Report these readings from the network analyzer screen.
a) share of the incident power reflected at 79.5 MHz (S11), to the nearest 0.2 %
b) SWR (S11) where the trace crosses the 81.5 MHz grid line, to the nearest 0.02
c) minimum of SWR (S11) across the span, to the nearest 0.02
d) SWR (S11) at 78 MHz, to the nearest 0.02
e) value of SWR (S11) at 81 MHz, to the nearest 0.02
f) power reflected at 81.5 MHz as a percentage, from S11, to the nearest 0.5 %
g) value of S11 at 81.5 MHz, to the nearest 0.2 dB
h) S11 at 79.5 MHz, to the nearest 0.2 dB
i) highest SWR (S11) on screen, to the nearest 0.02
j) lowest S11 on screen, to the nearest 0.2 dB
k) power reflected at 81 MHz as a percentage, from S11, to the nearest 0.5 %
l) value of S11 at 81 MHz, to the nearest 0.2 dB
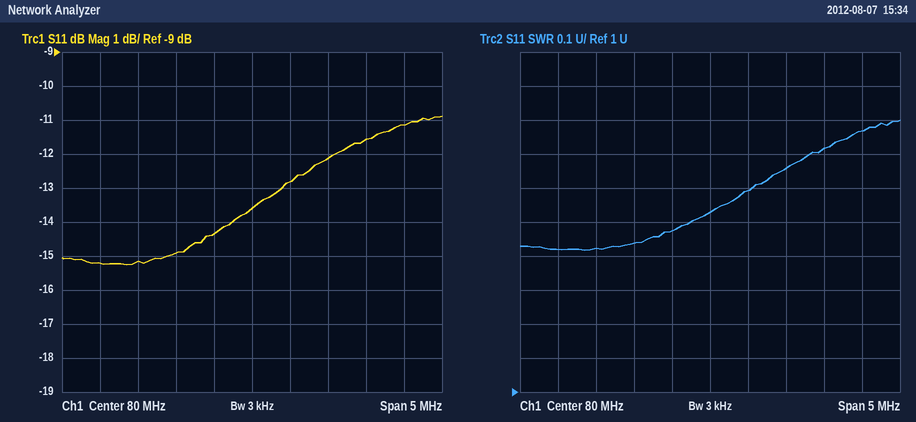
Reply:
3.6 %
1.72
1.42
1.42
1.66
7.0 %
-11.6 dB
-14.4 dB
1.80
-15.2 dB
6.0 %
-12.2 dB
